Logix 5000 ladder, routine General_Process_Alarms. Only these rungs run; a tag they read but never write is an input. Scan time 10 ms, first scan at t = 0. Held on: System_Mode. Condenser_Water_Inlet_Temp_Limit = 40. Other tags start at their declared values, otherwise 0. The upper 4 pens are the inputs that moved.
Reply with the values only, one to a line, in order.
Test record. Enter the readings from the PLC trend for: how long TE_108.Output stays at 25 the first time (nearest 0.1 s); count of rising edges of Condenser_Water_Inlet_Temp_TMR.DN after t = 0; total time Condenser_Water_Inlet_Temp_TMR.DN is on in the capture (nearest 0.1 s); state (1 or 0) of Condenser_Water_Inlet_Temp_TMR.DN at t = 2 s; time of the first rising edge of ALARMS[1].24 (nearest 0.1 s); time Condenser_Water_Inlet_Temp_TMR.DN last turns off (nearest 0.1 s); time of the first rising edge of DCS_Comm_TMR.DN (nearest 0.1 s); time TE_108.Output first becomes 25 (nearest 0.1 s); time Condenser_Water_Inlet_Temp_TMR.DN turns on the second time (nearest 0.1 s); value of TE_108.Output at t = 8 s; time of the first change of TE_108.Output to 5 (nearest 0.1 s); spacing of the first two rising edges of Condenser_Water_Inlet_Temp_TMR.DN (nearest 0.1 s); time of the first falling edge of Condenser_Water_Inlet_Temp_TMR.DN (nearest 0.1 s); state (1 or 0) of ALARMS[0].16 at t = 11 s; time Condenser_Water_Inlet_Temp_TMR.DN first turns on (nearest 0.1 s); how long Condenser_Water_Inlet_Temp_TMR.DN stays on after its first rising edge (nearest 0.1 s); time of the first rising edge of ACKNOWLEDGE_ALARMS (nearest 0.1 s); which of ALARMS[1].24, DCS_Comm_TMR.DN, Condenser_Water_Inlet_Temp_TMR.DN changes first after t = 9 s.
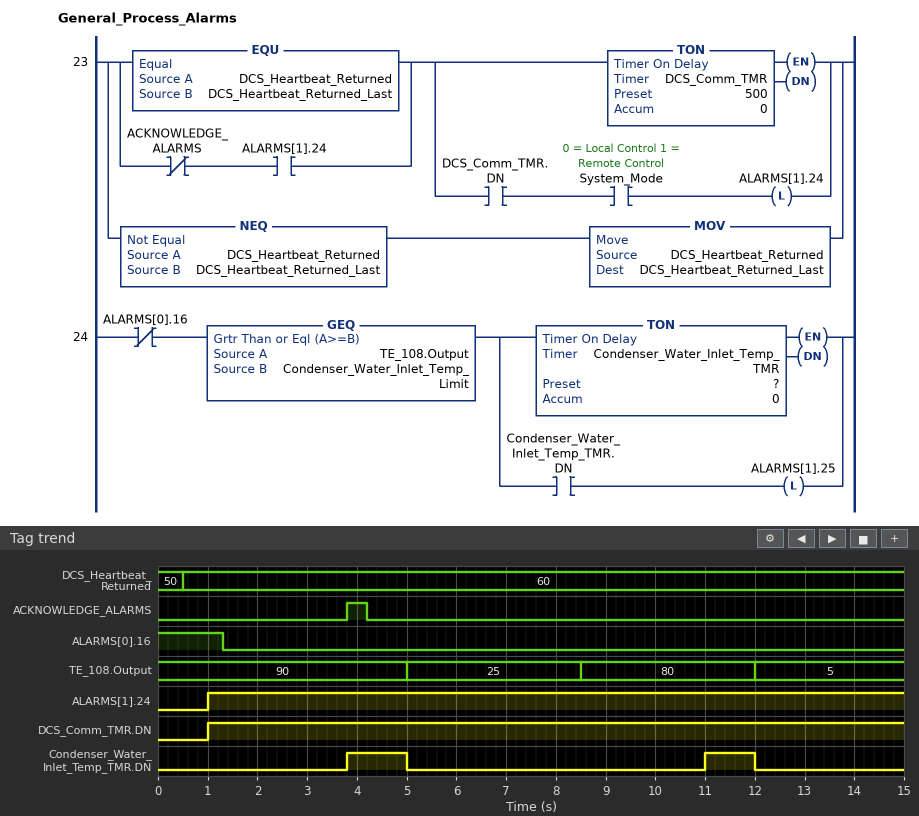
3.5 s
2
2.2 s
0
1.0 s
12.0 s
1.0 s
5.0 s
11.0 s
25
12.0 s
7.2 s
5.0 s
0
3.8 s
1.2 s
3.8 s
Condenser_Water_Inlet_Temp_TMR.DN
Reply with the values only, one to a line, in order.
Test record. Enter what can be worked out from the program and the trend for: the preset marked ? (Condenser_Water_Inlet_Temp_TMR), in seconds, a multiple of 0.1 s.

2.5 s
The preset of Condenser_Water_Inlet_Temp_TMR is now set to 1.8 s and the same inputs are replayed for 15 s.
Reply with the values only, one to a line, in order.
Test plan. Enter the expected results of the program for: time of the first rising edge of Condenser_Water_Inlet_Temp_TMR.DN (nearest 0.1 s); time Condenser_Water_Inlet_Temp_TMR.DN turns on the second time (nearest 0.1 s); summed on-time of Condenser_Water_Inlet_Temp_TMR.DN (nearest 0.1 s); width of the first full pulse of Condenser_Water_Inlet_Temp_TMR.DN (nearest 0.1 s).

3.1 s
10.3 s
3.6 s
1.9 s
